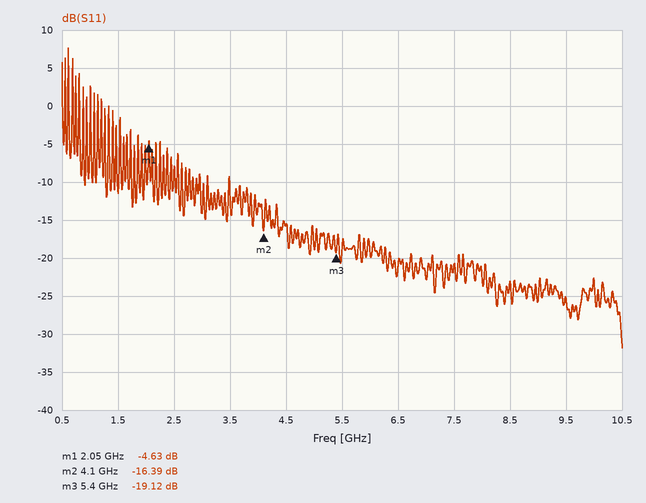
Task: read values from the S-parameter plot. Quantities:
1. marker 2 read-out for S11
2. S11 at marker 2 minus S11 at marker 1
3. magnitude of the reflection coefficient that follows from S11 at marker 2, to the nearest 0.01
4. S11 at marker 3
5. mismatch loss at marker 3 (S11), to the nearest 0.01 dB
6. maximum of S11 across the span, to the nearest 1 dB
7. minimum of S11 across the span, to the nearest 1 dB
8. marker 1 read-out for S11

-16.39 dB
-11.76 dB
0.15
-19.12 dB
0.05 dB
8 dB
-32 dB
-4.63 dB
